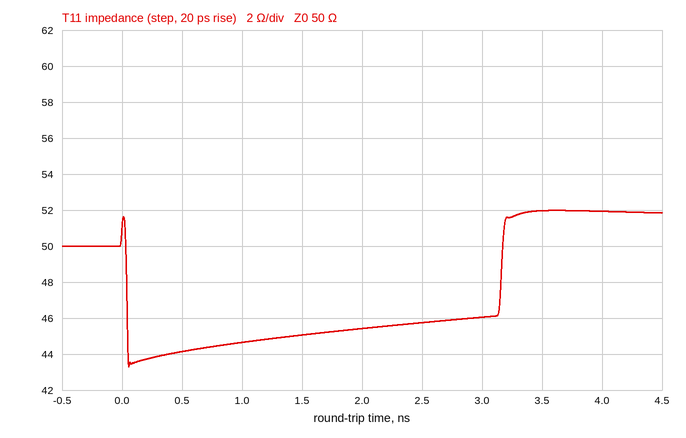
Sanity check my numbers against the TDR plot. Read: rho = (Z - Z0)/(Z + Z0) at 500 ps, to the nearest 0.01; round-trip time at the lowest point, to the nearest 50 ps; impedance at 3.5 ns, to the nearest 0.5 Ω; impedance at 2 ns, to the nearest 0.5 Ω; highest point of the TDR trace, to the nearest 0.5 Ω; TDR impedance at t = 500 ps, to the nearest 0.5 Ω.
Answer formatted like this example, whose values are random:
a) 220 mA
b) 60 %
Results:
a) -0.06
b) 50 ps
c) 52.0 Ω
d) 45.5 Ω
e) 52.0 Ω
f) 44.0 Ω
